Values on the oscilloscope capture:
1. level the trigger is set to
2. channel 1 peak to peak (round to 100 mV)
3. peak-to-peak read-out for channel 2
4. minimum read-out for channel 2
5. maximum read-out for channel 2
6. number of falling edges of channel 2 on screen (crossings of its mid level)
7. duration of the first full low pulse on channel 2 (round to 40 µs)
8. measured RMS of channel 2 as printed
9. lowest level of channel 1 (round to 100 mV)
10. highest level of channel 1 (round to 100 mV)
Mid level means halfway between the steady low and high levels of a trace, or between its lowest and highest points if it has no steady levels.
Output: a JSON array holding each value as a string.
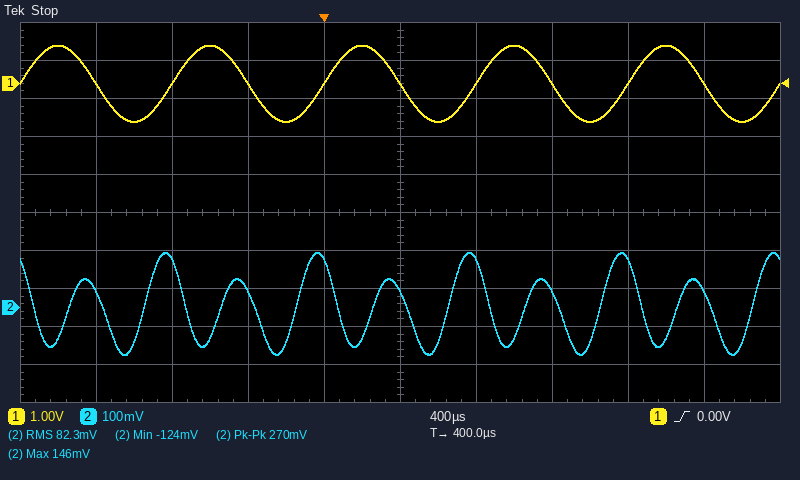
["0.00 V", "2.0 V", "270 mV", "-124 mV", "146 mV", "10", "200 µs", "82.3 mV", "-1.0 V", "1.0 V"]
